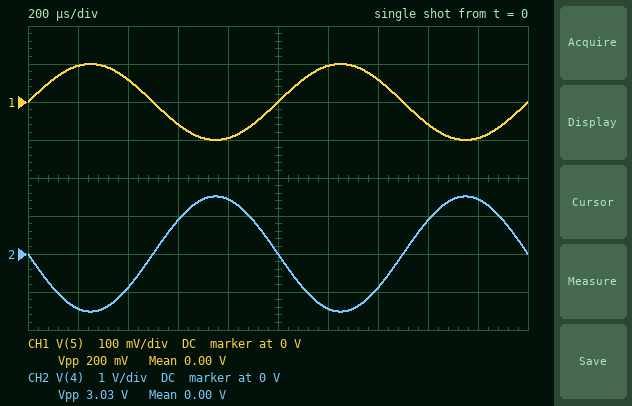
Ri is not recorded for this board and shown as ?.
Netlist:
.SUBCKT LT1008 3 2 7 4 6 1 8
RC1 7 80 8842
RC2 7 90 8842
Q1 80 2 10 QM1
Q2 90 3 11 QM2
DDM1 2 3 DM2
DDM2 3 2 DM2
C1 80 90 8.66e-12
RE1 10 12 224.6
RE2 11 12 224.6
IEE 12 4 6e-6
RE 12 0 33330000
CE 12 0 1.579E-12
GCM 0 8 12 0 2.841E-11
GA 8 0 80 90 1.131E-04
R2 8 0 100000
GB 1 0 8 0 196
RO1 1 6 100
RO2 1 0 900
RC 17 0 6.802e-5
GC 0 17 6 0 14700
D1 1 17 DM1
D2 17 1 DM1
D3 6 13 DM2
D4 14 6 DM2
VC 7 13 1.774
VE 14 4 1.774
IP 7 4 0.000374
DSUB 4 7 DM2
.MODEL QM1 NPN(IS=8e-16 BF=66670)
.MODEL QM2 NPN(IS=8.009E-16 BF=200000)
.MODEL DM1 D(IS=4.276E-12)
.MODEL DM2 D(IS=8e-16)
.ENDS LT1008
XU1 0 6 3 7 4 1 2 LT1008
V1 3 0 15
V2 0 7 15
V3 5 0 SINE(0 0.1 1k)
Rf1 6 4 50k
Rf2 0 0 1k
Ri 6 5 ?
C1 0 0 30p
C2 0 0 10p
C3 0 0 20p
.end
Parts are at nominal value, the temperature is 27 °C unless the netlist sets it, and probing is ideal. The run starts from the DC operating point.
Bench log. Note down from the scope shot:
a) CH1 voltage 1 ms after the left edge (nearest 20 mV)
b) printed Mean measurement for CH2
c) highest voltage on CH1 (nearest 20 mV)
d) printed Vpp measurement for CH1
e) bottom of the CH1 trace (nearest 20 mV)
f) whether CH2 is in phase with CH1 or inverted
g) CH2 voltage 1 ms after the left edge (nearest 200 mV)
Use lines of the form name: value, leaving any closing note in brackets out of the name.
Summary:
CH1 voltage 1 ms after the left edge: 0 V
printed Mean measurement for CH2: 0.00 V
highest voltage on CH1: 100 mV
printed Vpp measurement for CH1: 200 mV
bottom of the CH1 trace: -100 mV
whether CH2 is in phase with CH1 or inverted: inverted
CH2 voltage 1 ms after the left edge: 0 V
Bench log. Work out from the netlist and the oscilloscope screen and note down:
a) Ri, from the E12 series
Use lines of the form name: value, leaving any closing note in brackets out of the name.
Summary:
Ri, from the E12 series: 3.3 kΩ
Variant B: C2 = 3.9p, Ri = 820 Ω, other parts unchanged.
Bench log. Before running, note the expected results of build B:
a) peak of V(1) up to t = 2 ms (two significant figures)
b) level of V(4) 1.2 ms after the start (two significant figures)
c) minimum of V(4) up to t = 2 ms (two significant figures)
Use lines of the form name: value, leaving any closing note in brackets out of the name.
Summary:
peak of V(1) up to t = 2 ms: 6.1 V
level of V(4) 1.2 ms after the start: -5.8 V
minimum of V(4) up to t = 2 ms: -6.1 V
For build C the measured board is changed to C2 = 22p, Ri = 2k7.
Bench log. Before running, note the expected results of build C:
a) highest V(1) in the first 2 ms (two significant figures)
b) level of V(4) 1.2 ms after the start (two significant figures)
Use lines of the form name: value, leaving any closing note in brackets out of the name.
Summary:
highest V(1) in the first 2 ms: 1.9 V
level of V(4) 1.2 ms after the start: -1.8 V
